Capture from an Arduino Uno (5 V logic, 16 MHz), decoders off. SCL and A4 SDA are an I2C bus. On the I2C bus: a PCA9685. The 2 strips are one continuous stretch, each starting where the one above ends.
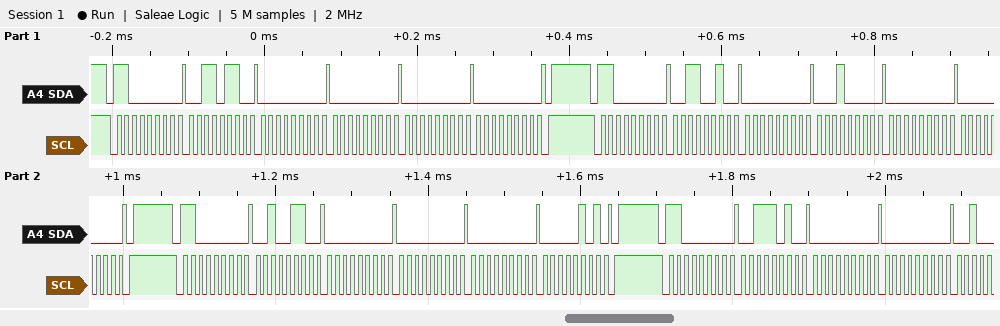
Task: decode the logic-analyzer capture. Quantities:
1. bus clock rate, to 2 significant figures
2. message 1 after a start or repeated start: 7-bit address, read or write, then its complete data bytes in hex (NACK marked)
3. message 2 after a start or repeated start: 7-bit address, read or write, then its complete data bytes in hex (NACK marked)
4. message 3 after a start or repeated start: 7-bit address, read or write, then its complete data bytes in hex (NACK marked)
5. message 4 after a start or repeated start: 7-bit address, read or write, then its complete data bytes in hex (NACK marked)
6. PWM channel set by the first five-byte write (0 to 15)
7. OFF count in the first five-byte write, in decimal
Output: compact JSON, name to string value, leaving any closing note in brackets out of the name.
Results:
{"bus clock rate, to 2 significant figures": "100 kHz", "message 1 after a start or repeated start: 7-bit address, read or write, then its complete data bytes in hex": "0x60 write: 36 00 00 00 00", "message 2 after a start or repeated start: 7-bit address, read or write, then its complete data bytes in hex": "0x60 write: 32 00 10 00 00", "message 3 after a start or repeated start: 7-bit address, read or write, then its complete data bytes in hex": "0x60 write: 26 00 00 00 05", "message 4 after a start or repeated start: 7-bit address, read or write, then its complete data bytes in hex": "0x60 write: 3A 00 00", "PWM channel set by the first five-byte write": "12", "OFF count in the first five-byte write, in decimal": "0"}
